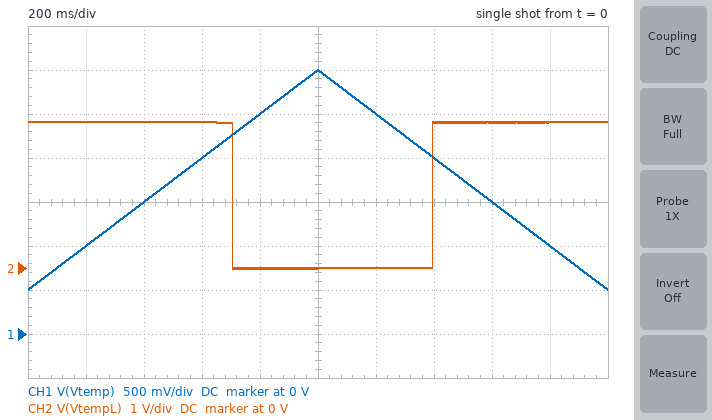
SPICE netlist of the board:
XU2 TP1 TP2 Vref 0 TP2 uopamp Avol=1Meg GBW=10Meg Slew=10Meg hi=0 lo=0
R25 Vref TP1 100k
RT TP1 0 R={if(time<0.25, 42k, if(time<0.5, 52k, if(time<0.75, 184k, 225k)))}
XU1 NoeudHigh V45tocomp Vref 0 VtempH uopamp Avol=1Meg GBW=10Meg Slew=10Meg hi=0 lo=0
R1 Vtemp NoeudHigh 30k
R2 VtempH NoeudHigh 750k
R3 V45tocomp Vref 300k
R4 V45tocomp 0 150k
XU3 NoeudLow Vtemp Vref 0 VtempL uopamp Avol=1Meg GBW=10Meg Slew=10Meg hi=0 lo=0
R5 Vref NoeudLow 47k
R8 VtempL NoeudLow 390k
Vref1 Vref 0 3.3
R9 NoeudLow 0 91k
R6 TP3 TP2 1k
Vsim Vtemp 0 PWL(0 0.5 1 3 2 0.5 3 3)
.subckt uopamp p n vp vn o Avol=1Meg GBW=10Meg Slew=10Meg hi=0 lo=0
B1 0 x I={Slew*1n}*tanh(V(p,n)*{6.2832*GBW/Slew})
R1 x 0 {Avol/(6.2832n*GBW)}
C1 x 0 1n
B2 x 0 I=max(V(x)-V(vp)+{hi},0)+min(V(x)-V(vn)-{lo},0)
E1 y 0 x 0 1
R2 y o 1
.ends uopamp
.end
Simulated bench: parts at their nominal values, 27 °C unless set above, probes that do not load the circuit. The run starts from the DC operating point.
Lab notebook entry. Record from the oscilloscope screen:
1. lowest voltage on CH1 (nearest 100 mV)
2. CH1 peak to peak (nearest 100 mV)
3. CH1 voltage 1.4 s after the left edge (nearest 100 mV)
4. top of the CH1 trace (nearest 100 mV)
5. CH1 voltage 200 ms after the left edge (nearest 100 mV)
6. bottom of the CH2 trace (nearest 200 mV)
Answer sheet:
500 mV
2.5 V
2.0 V
3.0 V
1.0 V
0 V
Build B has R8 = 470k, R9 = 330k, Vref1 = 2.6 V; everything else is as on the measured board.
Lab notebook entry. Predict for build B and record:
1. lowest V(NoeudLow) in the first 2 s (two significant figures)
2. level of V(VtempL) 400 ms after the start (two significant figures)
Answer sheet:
2.1 V
2.6 V
